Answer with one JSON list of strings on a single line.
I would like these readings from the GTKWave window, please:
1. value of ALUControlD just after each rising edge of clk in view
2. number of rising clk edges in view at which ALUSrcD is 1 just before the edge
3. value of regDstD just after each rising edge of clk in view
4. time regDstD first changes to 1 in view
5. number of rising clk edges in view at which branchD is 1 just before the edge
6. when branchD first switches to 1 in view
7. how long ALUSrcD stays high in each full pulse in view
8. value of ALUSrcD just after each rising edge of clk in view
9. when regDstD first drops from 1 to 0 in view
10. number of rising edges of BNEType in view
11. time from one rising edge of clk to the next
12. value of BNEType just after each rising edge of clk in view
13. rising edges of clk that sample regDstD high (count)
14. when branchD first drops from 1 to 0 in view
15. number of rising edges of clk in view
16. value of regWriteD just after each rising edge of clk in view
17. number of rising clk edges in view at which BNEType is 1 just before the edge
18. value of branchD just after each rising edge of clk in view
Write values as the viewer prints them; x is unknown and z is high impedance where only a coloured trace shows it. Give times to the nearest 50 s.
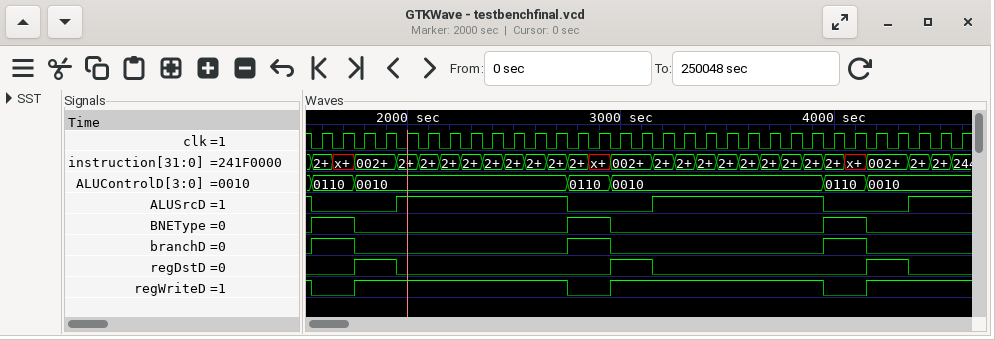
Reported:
["0110, 0110, 0010, 0010, 0010, 0010, 0010, 0010, 0010, 0010, 0010, 0010, 0110, 0110, 0010, 0010, 0010, 0010, 0010, 0010, 0010, 0010, 0010, 0010, 0110, 0110, 0010, 0010, 0010, 0010, 0010", "19", "0 0 1 1 0 0 0 0 0 0 0 0 0 0 1 1 0 0 0 0 0 0 0 0 0 0 1 1 0 0 0", "1750 s", "6", "1550 s", "800 s, 800 s", "0 0 0 0 1 1 1 1 1 1 1 1 0 0 0 0 1 1 1 1 1 1 1 1 0 0 0 0 1 1 1", "1950 s", "3", "100 s", "1 1 0 0 0 0 0 0 0 0 0 0 1 1 0 0 0 0 0 0 0 0 0 0 1 1 0 0 0 0 0", "6", "1750 s", "31", "0 0 1 1 1 1 1 1 1 1 1 1 0 0 1 1 1 1 1 1 1 1 1 1 0 0 1 1 1 1 1", "6", "1 1 0 0 0 0 0 0 0 0 0 0 1 1 0 0 0 0 0 0 0 0 0 0 1 1 0 0 0 0 0"]
